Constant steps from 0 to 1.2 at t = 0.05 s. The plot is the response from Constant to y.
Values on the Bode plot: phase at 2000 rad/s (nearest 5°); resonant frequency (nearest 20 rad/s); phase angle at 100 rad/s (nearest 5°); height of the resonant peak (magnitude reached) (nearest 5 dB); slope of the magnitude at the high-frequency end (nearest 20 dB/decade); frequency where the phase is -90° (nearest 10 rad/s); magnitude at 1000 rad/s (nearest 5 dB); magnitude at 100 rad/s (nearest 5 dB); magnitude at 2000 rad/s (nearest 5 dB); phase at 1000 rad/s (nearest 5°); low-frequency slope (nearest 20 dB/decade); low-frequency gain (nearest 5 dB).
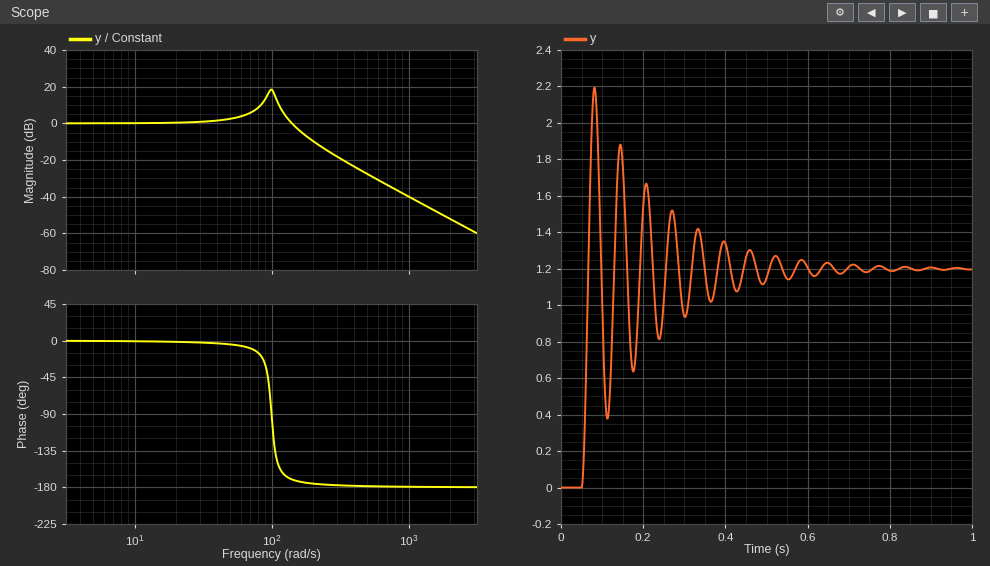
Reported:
-180°
100 rad/s
-90°
20 dB
-40 dB/decade
100 rad/s
-40 dB
20 dB
-50 dB
-180°
0 dB/decade
0 dB
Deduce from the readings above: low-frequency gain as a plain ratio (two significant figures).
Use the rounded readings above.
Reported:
1.0
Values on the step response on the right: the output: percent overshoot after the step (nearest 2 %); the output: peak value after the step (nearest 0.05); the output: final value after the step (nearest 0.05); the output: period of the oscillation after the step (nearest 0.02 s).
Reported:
82 %
2.20
1.20
0.06 s
